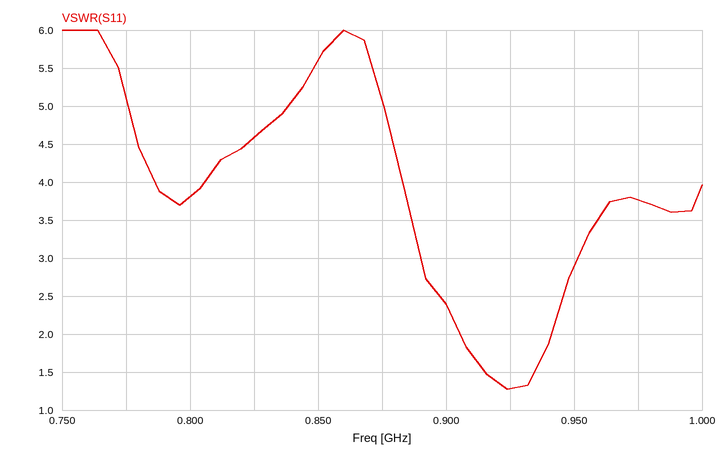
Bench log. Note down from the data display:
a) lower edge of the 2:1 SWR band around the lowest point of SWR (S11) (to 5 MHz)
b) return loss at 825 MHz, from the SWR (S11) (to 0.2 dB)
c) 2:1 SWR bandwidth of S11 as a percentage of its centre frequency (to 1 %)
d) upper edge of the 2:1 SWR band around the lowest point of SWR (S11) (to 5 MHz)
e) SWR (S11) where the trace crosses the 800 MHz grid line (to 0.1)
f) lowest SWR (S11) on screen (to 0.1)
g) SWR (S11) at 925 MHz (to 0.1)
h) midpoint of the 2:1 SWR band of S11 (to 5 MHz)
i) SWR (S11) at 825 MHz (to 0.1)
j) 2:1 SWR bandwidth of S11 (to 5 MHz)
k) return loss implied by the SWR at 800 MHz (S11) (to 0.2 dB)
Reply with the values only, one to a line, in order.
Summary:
905 MHz
3.8 dB
4 %
940 MHz
3.8
1.3
1.3
925 MHz
4.6
35 MHz
4.6 dB
